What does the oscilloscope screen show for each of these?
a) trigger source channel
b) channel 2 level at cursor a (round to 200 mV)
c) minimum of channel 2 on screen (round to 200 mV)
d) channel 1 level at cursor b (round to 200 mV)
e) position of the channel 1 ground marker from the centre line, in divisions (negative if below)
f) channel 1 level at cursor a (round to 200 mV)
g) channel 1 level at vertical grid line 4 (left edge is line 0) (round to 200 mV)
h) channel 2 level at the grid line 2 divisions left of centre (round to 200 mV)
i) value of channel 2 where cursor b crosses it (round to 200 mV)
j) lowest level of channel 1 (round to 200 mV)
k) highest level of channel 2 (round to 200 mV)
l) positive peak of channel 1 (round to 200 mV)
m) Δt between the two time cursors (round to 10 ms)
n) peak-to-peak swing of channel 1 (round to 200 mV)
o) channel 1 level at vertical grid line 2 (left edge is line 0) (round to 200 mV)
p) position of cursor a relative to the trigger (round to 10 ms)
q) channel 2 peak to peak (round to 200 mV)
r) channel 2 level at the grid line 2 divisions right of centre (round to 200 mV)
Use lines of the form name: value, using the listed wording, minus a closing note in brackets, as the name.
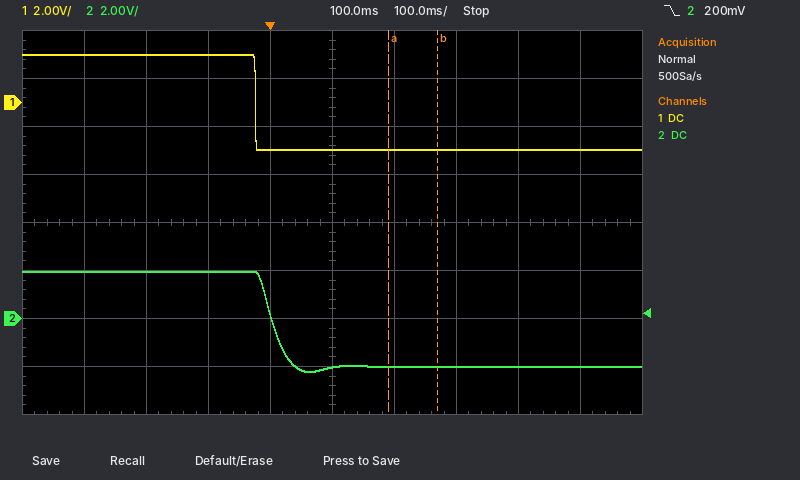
trigger source channel: channel 2
channel 2 level at cursor a: -2.0 V
minimum of channel 2 on screen: -2.2 V
channel 1 level at cursor b: -2.0 V
position of the channel 1 ground marker from the centre line, in divisions: +2.5 div
channel 1 level at cursor a: -2.0 V
channel 1 level at vertical grid line 4 (left edge is line 0): -2.0 V
channel 2 level at the grid line 2 divisions left of centre: 2.0 V
value of channel 2 where cursor b crosses it: -2.0 V
lowest level of channel 1: -2.0 V
highest level of channel 2: 2.0 V
positive peak of channel 1: 2.0 V
Δt between the two time cursors: 80 ms
peak-to-peak swing of channel 1: 4.0 V
channel 1 level at vertical grid line 2 (left edge is line 0): 2.0 V
position of cursor a relative to the trigger: +190 ms
channel 2 peak to peak: 4.2 V
channel 2 level at the grid line 2 divisions right of centre: -2.0 V
